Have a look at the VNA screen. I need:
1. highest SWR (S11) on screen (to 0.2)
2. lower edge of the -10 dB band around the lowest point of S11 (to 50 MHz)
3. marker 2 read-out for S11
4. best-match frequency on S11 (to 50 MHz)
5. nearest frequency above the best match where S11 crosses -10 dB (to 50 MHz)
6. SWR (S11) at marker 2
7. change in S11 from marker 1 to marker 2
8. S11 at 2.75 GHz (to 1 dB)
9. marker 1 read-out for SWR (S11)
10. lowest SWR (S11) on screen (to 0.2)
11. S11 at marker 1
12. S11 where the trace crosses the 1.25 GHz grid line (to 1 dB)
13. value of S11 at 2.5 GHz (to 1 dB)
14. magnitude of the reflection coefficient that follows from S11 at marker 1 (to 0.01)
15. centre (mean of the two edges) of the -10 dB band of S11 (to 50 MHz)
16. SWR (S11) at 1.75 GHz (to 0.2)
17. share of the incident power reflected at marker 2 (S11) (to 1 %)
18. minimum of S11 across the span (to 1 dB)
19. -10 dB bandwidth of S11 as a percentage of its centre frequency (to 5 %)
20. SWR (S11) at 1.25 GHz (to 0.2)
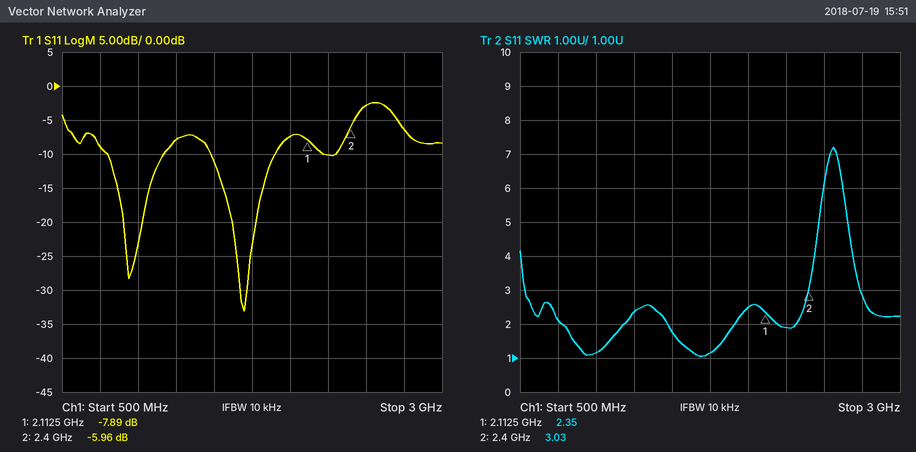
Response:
7.2
1.50 GHz
-5.96 dB
1.70 GHz
1.90 GHz
3.03
1.93 dB
-6 dB
2.35
1.0
-7.89 dB
-8 dB
-3 dB
0.40
1.70 GHz
1.2
25 %
-33 dB
25 %
2.4
